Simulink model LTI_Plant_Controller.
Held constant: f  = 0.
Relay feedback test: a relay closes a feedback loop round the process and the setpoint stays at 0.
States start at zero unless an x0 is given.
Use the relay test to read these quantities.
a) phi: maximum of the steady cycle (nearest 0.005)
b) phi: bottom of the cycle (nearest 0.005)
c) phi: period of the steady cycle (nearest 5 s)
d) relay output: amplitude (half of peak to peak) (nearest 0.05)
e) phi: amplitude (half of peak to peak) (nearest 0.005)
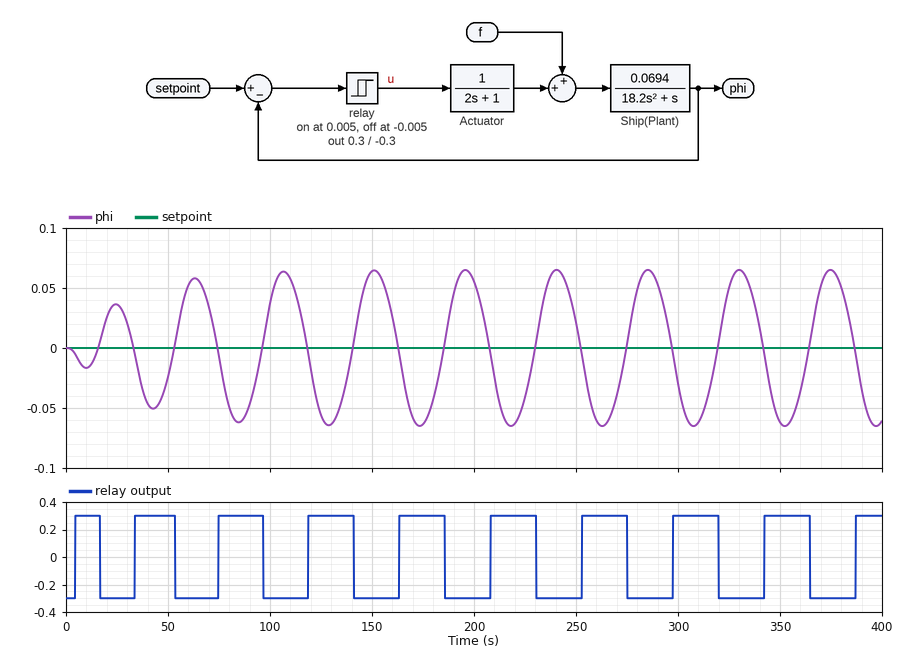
0.065
-0.065
45 s
0.30
0.065
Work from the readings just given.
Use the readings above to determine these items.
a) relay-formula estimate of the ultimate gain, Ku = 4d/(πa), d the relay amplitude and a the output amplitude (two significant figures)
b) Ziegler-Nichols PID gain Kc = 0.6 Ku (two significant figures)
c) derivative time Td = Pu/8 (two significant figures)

5.9
3.5
5.6 s
